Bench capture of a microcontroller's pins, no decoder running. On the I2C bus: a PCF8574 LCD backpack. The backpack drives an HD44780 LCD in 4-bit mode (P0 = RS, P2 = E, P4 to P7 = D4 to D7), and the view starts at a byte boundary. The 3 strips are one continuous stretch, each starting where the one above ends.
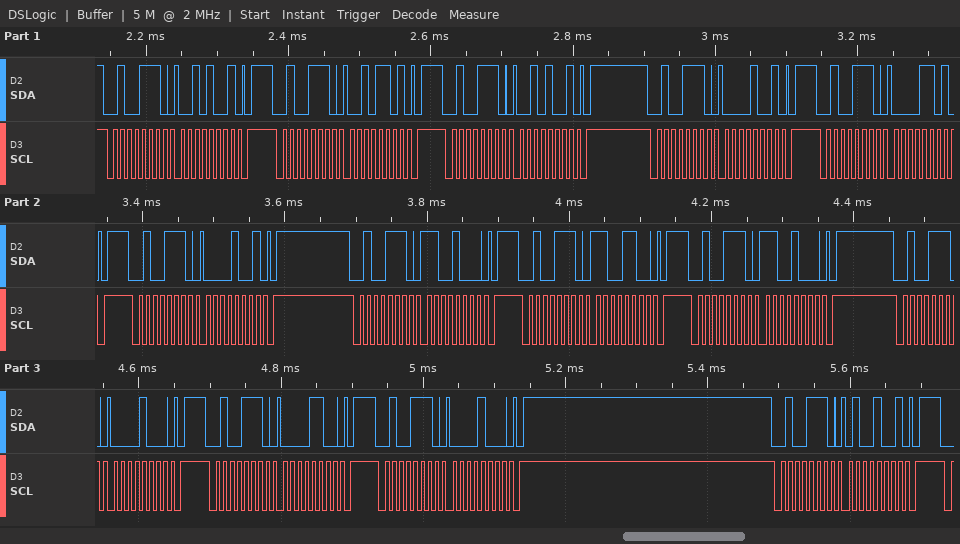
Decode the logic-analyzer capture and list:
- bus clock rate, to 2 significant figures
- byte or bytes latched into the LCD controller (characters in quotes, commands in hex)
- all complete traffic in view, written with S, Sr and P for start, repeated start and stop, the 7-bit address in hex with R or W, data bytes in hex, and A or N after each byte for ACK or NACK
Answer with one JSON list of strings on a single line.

["100 kHz", "' ' 0xC0", "S 27W A 29 A P S 27W A 2D A P S 27W A 29 A P S 27W A 09 A P S 27W A 0D A P S 27W A 09 A P S 27W A C8 A P S 27W A CC A P S 27W A C8 A P S 27W A 08 A P S 27W A 0C A P S 27W A 08 A P S 27W A 49 A P"]
